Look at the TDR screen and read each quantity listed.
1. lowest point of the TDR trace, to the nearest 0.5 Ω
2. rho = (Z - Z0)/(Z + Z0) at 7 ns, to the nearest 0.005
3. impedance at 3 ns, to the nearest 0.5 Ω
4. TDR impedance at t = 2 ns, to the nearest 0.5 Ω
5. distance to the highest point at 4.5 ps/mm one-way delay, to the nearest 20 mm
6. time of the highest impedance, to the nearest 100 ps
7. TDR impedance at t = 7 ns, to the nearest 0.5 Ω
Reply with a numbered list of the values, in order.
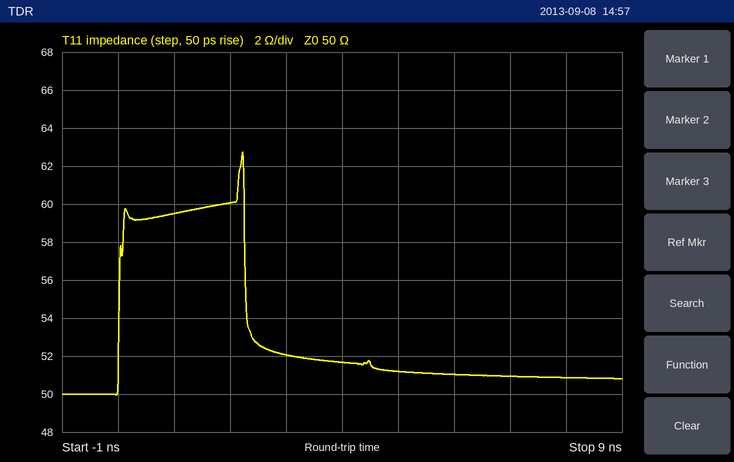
1. 50.0 Ω
2. +0.010
3. 52.0 Ω
4. 60.0 Ω
5. 240 mm
6. 2.2 ns
7. 51.0 Ω
